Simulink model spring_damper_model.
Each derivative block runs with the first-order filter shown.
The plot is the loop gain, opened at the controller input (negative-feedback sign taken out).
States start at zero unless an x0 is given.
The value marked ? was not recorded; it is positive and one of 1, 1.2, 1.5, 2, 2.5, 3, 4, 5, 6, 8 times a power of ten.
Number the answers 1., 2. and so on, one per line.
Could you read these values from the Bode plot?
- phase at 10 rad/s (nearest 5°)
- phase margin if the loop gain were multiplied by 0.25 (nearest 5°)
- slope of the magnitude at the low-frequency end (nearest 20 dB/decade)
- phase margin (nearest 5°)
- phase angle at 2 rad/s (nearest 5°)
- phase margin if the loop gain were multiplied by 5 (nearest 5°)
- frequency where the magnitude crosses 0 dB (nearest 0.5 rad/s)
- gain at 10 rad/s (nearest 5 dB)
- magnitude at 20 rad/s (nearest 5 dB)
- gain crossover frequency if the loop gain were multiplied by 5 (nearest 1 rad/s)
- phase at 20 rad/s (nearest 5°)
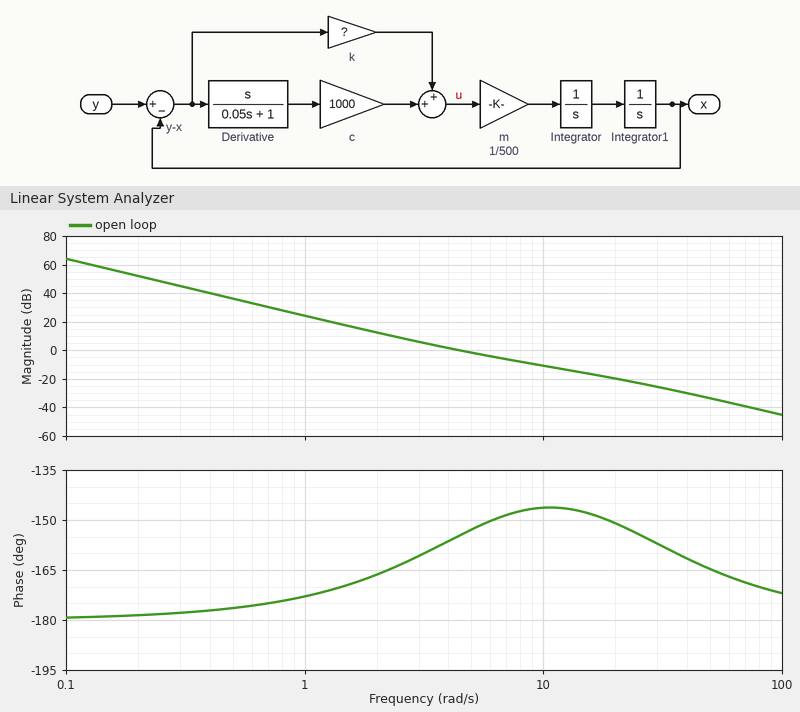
1. -145°
2. 15°
3. -40 dB/decade
4. 25°
5. -165°
6. 35°
7. 4.5 rad/s
8. -10 dB
9. -20 dB
10. 13 rad/s
11. -150°
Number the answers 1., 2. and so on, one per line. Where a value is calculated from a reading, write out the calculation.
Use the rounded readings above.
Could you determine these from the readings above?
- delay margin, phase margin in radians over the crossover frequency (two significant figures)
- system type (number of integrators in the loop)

1. 25 × π / 180 / 4.5 = 0.097 s
2. 2
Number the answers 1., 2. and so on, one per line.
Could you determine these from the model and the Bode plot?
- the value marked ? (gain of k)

1. 8000
